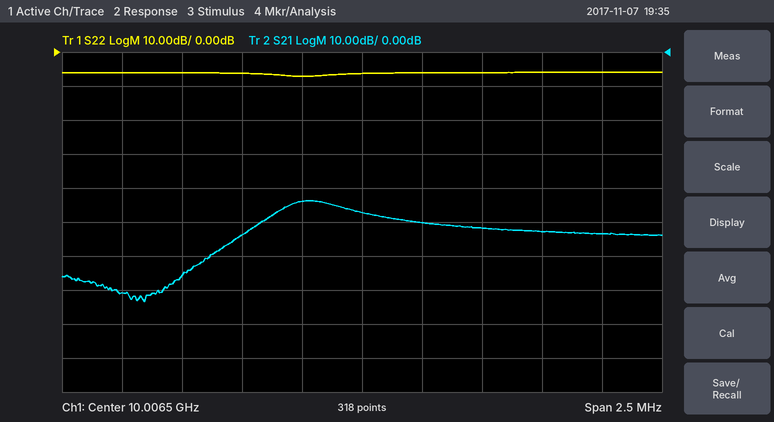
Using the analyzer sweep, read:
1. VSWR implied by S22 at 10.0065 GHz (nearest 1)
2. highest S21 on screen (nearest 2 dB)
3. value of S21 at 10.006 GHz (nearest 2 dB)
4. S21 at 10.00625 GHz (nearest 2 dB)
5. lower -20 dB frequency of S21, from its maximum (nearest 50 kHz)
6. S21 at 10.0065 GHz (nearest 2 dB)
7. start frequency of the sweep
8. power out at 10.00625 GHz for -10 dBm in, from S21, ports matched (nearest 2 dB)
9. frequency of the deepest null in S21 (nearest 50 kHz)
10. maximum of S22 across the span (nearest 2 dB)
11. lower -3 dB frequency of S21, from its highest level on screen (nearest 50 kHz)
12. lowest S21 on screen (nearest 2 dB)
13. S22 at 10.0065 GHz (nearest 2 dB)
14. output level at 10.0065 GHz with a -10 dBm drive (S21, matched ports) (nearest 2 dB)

3
-44 dB
-54 dB
-44 dB
10.00580 GHz
-48 dB
10.00525 GHz
-54 dBm
10.00560 GHz
-6 dB
10.00615 GHz
-74 dB
-6 dB
-58 dBm
